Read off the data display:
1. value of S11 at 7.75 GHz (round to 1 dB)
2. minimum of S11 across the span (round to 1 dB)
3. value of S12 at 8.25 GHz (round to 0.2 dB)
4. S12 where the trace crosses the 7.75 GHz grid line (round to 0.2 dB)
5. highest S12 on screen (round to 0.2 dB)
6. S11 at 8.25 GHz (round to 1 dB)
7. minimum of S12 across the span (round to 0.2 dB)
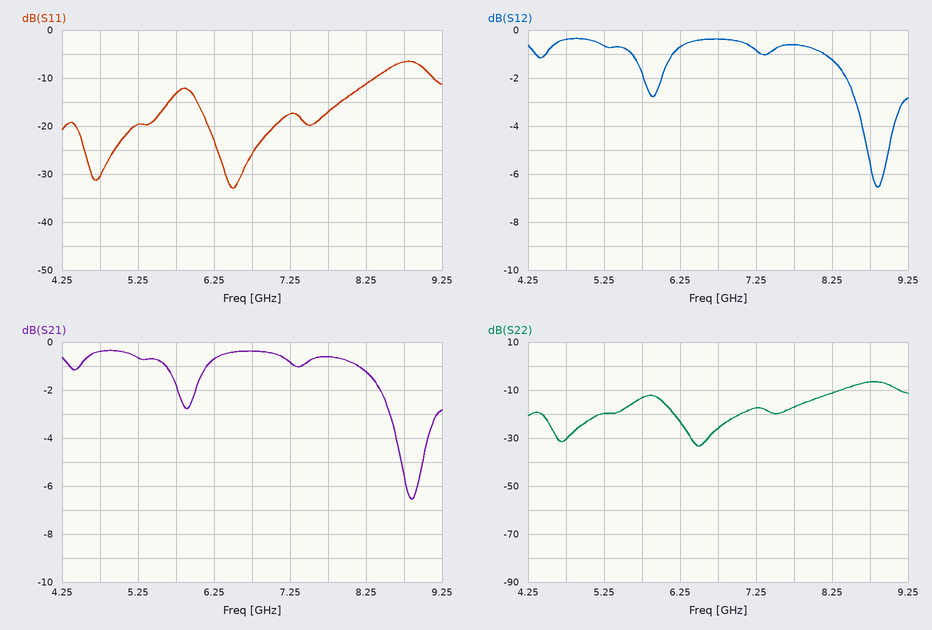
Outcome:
-17 dB
-33 dB
-1.2 dB
-0.6 dB
-0.4 dB
-11 dB
-6.6 dB
